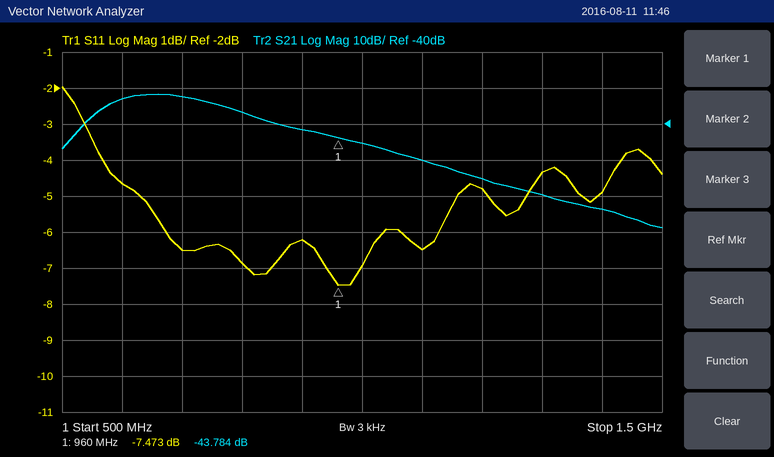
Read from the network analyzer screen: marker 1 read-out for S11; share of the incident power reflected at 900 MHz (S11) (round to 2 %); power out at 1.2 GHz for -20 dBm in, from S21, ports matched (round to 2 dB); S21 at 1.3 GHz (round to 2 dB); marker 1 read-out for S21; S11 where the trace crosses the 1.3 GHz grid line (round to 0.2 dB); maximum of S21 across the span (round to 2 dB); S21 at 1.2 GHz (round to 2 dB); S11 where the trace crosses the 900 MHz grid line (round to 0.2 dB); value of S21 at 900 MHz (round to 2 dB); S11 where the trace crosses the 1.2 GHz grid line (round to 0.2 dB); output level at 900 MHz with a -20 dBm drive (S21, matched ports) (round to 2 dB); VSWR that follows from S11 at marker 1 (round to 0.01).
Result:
-7.473 dB
24 %
-76 dBm
-60 dB
-43.784 dB
-4.4 dB
-32 dB
-56 dB
-6.2 dB
-42 dB
-4.8 dB
-62 dBm
2.47
